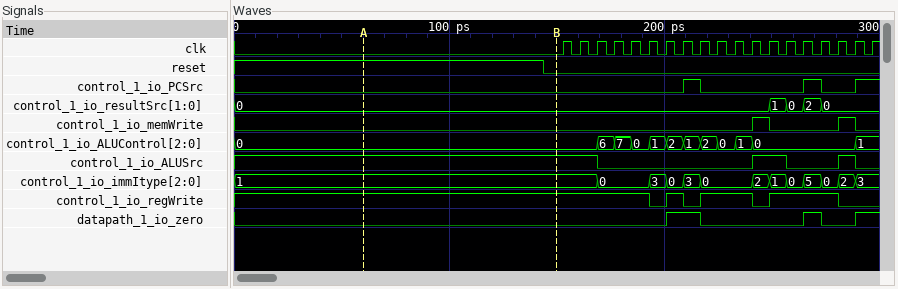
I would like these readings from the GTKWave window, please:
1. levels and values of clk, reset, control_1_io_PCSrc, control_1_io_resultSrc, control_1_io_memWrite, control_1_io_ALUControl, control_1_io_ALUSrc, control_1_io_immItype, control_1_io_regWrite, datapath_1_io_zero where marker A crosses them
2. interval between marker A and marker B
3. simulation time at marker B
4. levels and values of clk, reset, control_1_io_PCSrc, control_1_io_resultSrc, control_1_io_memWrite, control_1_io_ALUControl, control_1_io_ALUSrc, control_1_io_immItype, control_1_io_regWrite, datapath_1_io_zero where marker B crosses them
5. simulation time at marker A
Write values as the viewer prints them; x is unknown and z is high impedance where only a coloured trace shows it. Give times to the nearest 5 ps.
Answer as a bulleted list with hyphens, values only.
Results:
- clk=0, reset=1, control_1_io_PCSrc=0, control_1_io_resultSrc=0, control_1_io_memWrite=0, control_1_io_ALUControl=0, control_1_io_ALUSrc=1, control_1_io_immItype=1, control_1_io_regWrite=1, datapath_1_io_zero=0
- 90 ps
- 150 ps
- clk=0, reset=0, control_1_io_PCSrc=0, control_1_io_resultSrc=0, control_1_io_memWrite=0, control_1_io_ALUControl=0, control_1_io_ALUSrc=1, control_1_io_immItype=1, control_1_io_regWrite=1, datapath_1_io_zero=0
- 60 ps
